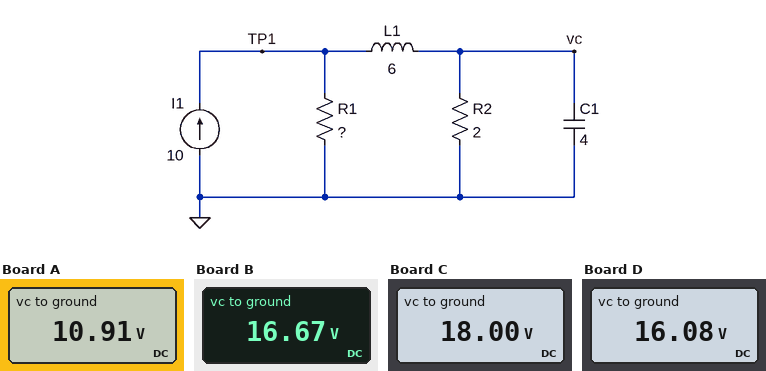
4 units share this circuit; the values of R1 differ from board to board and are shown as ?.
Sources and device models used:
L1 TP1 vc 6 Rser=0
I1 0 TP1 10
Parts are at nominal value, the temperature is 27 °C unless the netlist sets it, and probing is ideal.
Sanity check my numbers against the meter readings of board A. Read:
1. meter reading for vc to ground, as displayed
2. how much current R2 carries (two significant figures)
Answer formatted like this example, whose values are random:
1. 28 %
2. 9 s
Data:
1. 10.91 V
2. 5.5 A
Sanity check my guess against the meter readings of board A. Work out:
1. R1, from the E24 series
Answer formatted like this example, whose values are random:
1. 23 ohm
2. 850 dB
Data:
1. 2.4 Ω
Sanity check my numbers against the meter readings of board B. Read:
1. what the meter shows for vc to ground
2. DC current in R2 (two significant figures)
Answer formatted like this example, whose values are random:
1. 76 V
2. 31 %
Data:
1. 16.67 V
2. 8.3 A
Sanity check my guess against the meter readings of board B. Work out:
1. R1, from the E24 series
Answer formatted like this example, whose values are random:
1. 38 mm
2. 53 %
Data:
1. 10 Ω
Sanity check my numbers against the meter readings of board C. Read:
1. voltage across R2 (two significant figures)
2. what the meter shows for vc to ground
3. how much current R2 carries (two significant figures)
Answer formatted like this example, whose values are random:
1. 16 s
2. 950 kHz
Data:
1. 18 V
2. 18.00 V
3. 9.0 A
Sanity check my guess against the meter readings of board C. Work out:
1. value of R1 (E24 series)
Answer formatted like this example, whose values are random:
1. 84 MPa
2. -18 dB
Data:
1. 18 Ω
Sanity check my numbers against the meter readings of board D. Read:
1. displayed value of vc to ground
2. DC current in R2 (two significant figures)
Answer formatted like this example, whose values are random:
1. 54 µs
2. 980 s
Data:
1. 16.08 V
2. 8.0 A
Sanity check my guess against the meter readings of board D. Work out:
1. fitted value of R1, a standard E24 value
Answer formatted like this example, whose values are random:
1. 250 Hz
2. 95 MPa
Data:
1. 8.2 Ω
